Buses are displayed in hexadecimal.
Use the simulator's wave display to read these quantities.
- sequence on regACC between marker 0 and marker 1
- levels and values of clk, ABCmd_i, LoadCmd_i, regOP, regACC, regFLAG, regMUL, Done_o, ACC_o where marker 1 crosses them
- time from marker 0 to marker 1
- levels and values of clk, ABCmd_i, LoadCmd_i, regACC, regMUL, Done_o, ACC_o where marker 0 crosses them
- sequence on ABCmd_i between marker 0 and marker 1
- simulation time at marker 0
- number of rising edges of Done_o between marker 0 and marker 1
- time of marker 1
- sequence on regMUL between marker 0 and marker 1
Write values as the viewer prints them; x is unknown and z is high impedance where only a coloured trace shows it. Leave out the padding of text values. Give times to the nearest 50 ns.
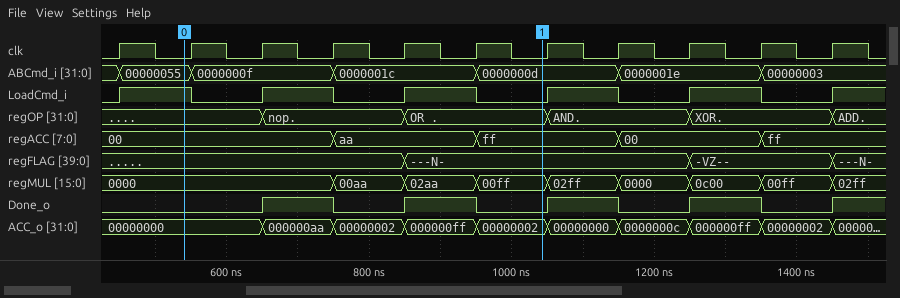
00, aa, ff
clk=0, ABCmd_i=0000000d, LoadCmd_i=0, regOP=OR, regACC=ff, regFLAG=---N-, regMUL=00ff, Done_o=0, ACC_o=00000002
500 ns
clk=0, ABCmd_i=00000055, LoadCmd_i=1, regACC=00, regMUL=0000, Done_o=0, ACC_o=00000000
00000055, 0000000f, 0000001c, 0000000d
550 ns
2
1050 ns
0000, 00aa, 02aa, 00ff
